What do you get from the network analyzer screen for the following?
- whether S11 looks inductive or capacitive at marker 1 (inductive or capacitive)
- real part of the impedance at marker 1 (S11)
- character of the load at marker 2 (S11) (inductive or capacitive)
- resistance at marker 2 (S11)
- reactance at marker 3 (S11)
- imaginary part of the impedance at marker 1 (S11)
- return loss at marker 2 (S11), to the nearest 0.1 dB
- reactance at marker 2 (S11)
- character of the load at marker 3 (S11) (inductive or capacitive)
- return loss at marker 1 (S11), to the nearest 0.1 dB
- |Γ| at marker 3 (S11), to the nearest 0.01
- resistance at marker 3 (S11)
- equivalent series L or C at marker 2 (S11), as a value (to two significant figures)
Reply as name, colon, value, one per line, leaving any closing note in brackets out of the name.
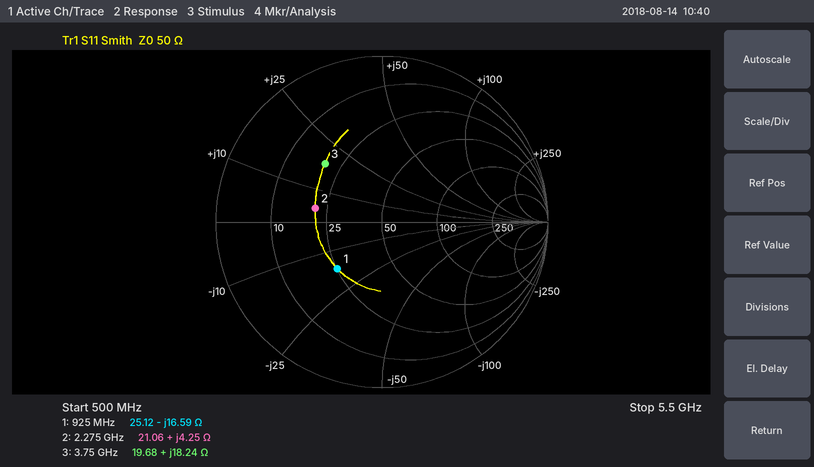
whether S11 looks inductive or capacitive at marker 1: capacitive
real part of the impedance at marker 1: 25.12 Ω
character of the load at marker 2 (S11): inductive
resistance at marker 2: 21.06 Ω
reactance at marker 3: +18.24 Ω
imaginary part of the impedance at marker 1: -16.59 Ω
return loss at marker 2 (S11), to the nearest 0.1 dB: 7.7 dB
reactance at marker 2: +4.25 Ω
character of the load at marker 3 (S11): inductive
return loss at marker 1 (S11), to the nearest 0.1 dB: 8.2 dB
|Γ| at marker 3 (S11), to the nearest 0.01: 0.49
resistance at marker 3: 19.68 Ω
equivalent series L or C at marker 2 (S11), as a value: 300 pH
